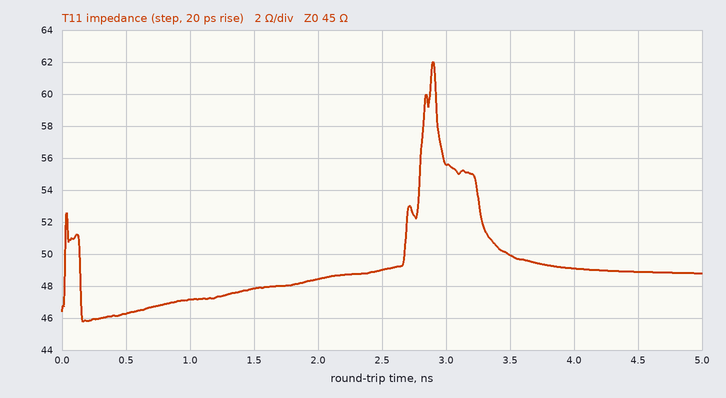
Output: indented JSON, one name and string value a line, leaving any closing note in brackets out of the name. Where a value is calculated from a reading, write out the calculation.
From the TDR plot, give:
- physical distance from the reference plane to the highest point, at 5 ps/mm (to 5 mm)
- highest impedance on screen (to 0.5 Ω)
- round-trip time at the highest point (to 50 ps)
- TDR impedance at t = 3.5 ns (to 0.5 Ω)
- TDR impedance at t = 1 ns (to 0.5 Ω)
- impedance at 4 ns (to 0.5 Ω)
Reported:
{
  "physical distance from the reference plane to the highest point, at 5 ps/mm": "2.90 ns / 2 / 5 ps/mm ≈ 290 mm",
  "highest impedance on screen": "62.0 Ω",
  "round-trip time at the highest point": "2.90 ns",
  "TDR impedance at t = 3.5 ns": "50.0 Ω",
  "TDR impedance at t = 1 ns": "47.0 Ω",
  "impedance at 4 ns": "49.0 Ω"
}
